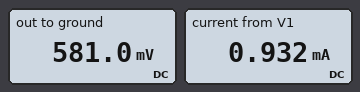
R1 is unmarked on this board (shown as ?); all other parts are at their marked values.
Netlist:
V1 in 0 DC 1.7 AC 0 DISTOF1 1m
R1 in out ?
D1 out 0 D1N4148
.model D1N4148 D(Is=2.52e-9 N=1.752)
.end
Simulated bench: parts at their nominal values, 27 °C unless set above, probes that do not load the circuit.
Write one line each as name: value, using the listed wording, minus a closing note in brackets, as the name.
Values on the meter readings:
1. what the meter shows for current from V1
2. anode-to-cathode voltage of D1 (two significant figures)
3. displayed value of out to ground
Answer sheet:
what the meter shows for current from V1: 0.932 mA
anode-to-cathode voltage of D1: 580 mV
displayed value of out to ground: 581.0 mV
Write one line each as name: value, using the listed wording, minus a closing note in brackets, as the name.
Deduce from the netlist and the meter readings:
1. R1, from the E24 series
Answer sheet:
R1, from the E24 series: 1.2 kΩ
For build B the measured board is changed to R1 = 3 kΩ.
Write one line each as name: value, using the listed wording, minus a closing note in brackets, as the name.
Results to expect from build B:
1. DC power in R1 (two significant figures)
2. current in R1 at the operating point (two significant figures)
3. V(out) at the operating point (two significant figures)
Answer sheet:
DC power in R1: 450 µW
current in R1 at the operating point: 390 µA
V(out) at the operating point: 540 mV
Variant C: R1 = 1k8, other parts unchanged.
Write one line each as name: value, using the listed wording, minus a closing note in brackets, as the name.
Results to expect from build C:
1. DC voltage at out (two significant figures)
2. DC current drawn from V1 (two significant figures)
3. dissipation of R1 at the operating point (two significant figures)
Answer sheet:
DC voltage at out: 560 mV
DC current drawn from V1: 630 µA
dissipation of R1 at the operating point: 720 µW
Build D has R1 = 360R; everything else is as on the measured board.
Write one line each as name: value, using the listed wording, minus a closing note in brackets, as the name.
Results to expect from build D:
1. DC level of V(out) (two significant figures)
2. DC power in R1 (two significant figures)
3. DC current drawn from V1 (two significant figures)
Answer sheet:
DC level of V(out): 630 mV
DC power in R1: 3.2 mW
DC current drawn from V1: 3.0 mA
